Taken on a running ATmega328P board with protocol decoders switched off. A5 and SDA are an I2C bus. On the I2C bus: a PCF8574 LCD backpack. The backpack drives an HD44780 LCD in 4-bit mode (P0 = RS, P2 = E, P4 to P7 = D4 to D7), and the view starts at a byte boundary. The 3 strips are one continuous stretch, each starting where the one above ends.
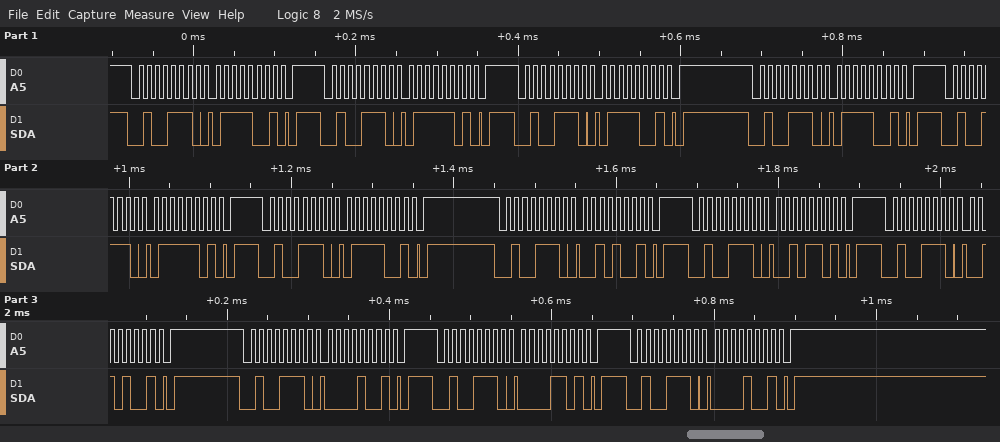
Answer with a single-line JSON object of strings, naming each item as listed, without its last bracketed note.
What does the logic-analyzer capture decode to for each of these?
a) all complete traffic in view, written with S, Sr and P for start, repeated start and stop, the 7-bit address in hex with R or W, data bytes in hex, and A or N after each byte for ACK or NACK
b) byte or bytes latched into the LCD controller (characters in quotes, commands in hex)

{"all complete traffic in view, written with S, Sr and P for start, repeated start and stop, the 7-bit address in hex with R or W, data bytes in hex, and A or N after each byte for ACK or NACK": "S 27W A 79 A P S 27W A 7D A P S 27W A 79 A P S 27W A 79 A P S 27W A 7D A P S 27W A 79 A P S 27W A 29 A P S 27W A 2D A P S 27W A 29 A P S 27W A 09 A P S 27W A 0D A P S 27W A 09 A P", "byte or bytes latched into the LCD controller": "'w' ' '"}
